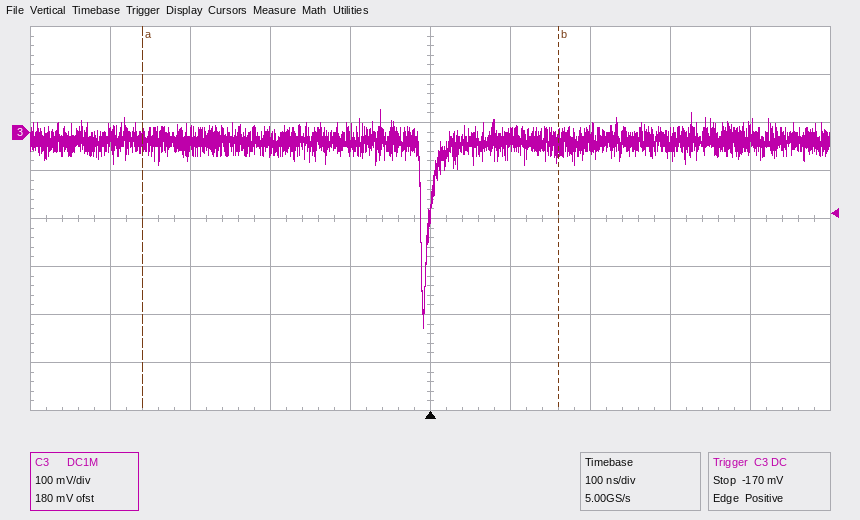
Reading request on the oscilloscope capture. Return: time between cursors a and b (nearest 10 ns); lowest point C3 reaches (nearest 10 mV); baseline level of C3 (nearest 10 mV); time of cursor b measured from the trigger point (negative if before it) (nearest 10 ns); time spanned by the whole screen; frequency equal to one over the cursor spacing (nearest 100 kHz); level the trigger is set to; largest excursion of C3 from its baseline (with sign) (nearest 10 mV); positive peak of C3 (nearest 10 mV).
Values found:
520 ns
-410 mV
-20 mV
+160 ns
1 µs
1.9 MHz
-170 mV
-390 mV
50 mV
